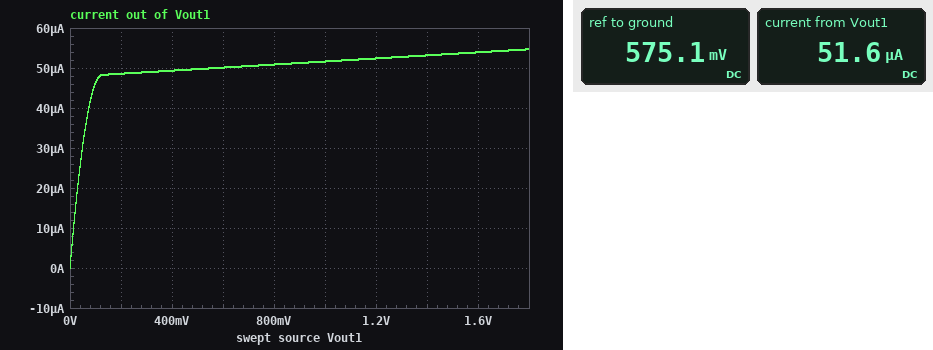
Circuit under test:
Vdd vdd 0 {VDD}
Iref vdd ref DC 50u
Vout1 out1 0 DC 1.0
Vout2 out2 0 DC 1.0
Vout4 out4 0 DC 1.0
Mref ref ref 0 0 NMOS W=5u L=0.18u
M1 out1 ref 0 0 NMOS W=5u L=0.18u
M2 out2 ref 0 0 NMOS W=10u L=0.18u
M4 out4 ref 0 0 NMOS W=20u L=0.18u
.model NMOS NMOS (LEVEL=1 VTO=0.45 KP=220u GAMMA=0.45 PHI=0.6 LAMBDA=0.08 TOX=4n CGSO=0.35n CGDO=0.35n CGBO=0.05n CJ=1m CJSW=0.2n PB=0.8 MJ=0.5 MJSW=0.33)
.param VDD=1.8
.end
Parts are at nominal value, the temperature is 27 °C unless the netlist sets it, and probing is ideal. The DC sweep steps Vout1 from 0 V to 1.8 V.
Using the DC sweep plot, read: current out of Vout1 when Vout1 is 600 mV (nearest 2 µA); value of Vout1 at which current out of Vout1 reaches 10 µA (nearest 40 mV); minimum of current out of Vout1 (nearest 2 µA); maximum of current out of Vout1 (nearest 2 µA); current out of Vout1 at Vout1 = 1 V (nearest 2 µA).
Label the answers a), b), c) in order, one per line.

a) 50 µA
b) 0 V
c) 0 A
d) 54 µA
e) 52 µA
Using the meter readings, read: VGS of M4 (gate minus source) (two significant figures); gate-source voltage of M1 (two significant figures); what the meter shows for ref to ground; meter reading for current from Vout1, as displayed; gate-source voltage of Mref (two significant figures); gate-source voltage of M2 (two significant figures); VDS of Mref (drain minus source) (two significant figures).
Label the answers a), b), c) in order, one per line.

a) 580 mV
b) 580 mV
c) 575.1 mV
d) 51.6 µA
e) 580 mV
f) 580 mV
g) 580 mV
